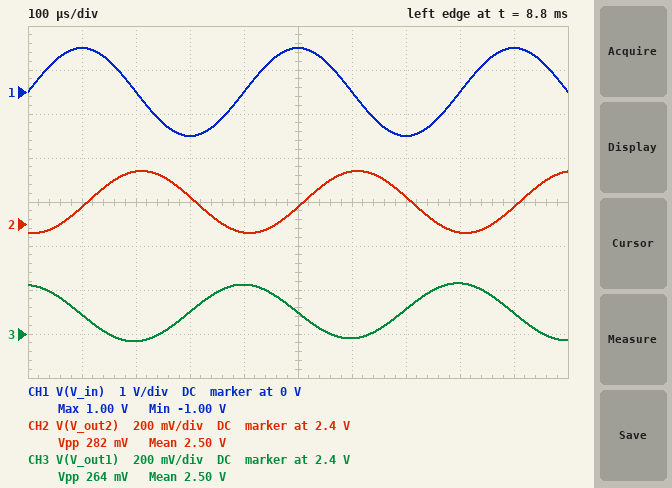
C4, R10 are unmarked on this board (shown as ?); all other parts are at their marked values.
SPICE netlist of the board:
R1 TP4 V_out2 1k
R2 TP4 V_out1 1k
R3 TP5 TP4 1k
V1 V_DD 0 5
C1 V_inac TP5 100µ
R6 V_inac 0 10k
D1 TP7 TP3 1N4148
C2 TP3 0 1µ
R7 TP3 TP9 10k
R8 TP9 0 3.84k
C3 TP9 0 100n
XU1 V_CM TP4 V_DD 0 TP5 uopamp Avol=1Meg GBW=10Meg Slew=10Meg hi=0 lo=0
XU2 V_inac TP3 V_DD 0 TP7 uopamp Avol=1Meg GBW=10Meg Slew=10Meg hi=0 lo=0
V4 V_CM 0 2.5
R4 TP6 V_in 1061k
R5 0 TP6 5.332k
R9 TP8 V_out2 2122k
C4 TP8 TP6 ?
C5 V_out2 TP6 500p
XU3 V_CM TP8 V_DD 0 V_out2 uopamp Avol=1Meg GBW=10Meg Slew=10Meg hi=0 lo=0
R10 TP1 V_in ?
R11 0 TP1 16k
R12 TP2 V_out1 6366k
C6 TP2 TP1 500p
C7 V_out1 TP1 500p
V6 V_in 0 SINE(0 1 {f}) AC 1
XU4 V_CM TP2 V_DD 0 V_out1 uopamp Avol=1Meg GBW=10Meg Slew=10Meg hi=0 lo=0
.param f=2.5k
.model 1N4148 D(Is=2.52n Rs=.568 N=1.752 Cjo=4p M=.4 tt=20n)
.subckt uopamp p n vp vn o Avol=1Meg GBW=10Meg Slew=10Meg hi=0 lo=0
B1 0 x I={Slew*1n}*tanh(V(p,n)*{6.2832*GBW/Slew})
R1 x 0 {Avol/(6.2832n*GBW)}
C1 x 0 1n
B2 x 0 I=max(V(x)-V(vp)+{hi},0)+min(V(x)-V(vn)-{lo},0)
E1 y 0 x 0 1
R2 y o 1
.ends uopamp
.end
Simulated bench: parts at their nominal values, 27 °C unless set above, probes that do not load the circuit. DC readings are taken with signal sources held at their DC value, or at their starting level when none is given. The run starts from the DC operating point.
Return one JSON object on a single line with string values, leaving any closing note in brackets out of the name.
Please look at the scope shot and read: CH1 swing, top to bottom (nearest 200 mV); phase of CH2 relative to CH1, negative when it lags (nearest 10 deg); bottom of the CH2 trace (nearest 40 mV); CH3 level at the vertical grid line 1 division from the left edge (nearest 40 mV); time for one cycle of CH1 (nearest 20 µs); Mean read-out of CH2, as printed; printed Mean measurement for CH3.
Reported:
{"CH1 swing, top to bottom": "2.0 V", "phase of CH2 relative to CH1, negative when it lags": "-100 deg", "bottom of the CH2 trace": "2.36 V", "CH3 level at the vertical grid line 1 division from the left edge": "2.48 V", "time for one cycle of CH1": "400 µs", "Mean read-out of CH2, as printed": "2.50 V", "printed Mean measurement for CH3": "2.50 V"}
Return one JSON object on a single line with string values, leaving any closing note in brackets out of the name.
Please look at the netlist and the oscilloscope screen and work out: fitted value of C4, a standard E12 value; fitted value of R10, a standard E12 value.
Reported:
{"fitted value of C4, a standard E12 value": "390 pF", "fitted value of R10, a standard E12 value": "1.2 MΩ"}
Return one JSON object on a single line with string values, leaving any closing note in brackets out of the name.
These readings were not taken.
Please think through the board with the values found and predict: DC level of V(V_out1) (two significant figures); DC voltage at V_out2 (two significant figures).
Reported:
{"DC level of V(V_out1)": "2.5 V", "DC voltage at V_out2": "2.5 V"}
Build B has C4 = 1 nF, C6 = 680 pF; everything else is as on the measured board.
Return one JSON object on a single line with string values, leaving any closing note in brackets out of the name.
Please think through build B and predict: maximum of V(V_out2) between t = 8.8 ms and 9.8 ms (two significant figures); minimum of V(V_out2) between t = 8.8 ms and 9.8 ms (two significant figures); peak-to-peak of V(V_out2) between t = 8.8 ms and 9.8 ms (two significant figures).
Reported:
{"maximum of V(V_out2) between t = 8.8 ms and 9.8 ms": "2.9 V", "minimum of V(V_out2) between t = 8.8 ms and 9.8 ms": "2.1 V", "peak-to-peak of V(V_out2) between t = 8.8 ms and 9.8 ms": "800 mV"}
